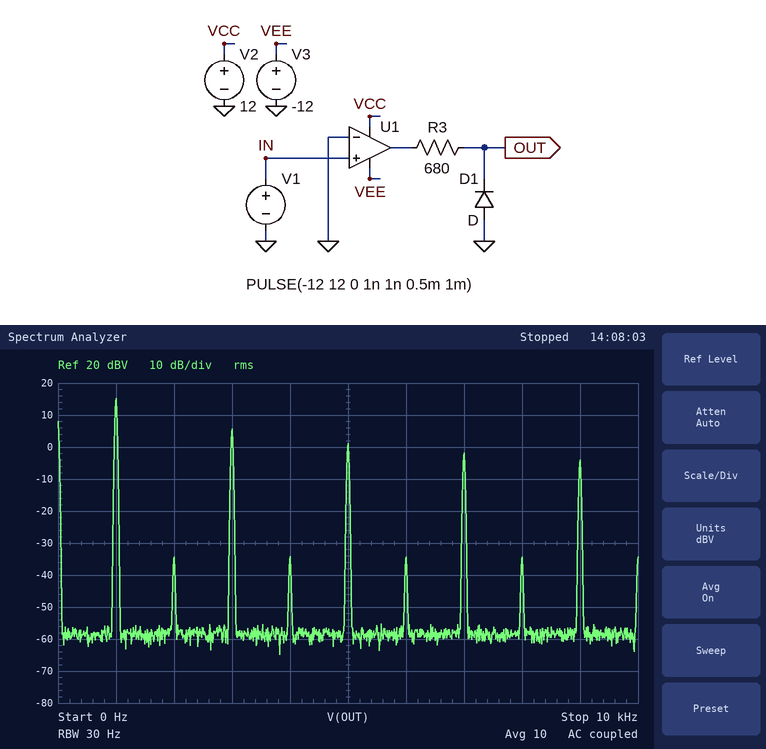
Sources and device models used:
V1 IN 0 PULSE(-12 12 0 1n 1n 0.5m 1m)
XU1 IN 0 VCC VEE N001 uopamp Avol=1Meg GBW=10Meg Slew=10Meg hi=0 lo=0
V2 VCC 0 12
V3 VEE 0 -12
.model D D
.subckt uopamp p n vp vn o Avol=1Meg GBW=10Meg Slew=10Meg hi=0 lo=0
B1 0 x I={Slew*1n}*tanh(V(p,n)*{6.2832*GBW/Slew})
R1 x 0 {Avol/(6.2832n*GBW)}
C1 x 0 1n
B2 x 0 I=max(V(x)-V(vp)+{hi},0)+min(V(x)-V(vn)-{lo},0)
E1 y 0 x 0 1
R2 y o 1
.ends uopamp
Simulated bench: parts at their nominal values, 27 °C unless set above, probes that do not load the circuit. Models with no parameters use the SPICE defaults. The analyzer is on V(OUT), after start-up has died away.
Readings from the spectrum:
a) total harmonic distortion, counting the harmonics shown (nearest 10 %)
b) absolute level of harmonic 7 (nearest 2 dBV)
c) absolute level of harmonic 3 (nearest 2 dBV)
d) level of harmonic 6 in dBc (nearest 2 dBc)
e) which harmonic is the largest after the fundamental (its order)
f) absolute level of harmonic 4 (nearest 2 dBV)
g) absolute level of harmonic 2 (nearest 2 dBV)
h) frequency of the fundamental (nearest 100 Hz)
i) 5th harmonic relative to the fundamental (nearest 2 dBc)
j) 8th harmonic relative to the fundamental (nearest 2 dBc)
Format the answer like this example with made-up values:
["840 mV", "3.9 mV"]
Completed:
["40 %", "-2 dBV", "6 dBV", "-50 dBc", "3", "-34 dBV", "-34 dBV", "1.0 kHz", "-14 dBc", "-50 dBc"]
